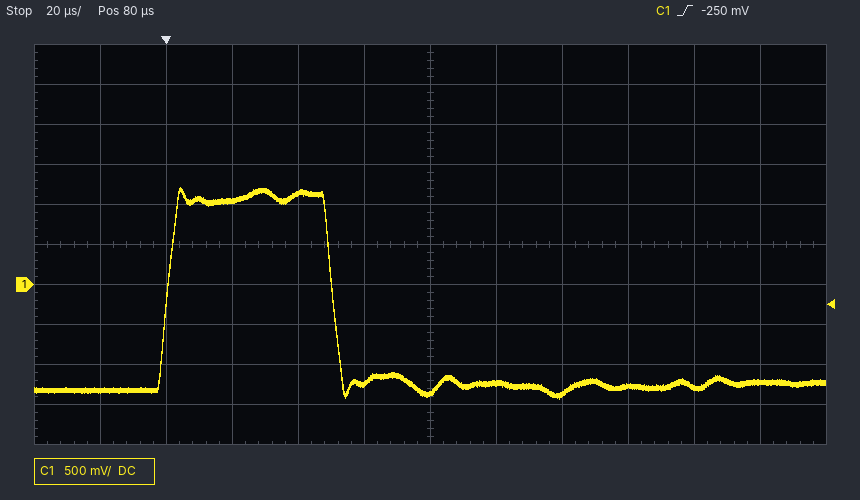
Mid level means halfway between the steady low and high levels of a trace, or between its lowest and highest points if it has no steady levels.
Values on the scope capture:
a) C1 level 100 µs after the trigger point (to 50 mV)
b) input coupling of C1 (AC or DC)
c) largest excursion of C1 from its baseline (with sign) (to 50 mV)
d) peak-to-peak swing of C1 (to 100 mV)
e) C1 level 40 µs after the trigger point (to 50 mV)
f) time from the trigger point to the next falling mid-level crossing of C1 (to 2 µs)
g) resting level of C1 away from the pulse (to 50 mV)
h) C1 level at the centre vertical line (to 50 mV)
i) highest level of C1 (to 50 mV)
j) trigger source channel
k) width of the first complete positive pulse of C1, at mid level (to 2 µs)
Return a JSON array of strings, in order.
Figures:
["-1.25 V", "DC", "+2.45 V", "2.60 V", "1.15 V", "50 µs", "-1.25 V", "-1.35 V", "1.20 V", "C1", "50 µs"]
